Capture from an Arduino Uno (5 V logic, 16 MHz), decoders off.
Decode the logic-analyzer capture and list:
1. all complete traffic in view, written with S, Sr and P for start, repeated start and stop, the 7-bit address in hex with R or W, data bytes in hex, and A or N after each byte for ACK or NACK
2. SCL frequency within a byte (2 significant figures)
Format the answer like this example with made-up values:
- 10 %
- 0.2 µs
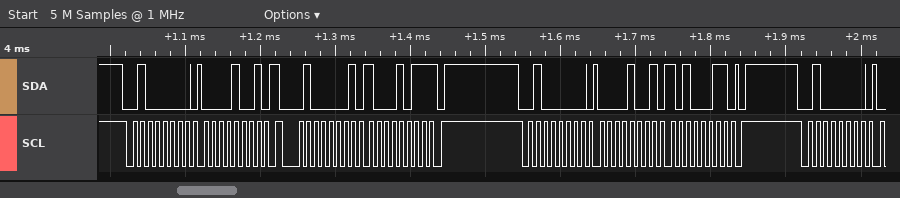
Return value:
- S 20W A 09 A Sr 20R A 8B N P S 20W A 09 A A3 A P S 20W A
- 100 kHz
